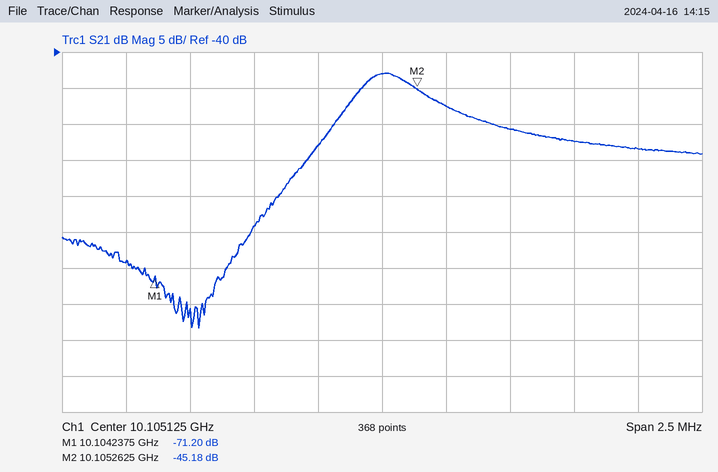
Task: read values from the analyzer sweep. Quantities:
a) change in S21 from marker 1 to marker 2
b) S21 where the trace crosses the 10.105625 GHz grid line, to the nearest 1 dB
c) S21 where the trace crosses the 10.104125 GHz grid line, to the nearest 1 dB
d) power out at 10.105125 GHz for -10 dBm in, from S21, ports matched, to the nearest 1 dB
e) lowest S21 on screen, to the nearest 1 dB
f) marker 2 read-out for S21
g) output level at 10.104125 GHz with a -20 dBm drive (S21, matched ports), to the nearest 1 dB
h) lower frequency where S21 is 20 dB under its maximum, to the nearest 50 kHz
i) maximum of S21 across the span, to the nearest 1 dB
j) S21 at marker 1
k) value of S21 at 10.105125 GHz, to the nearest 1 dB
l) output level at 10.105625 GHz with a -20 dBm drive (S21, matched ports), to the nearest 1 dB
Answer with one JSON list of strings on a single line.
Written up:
["26.02 dB", "-51 dB", "-69 dB", "-53 dBm", "-78 dB", "-45.18 dB", "-89 dBm", "10.10465 GHz", "-43 dB", "-71.20 dB", "-43 dB", "-71 dBm"]
